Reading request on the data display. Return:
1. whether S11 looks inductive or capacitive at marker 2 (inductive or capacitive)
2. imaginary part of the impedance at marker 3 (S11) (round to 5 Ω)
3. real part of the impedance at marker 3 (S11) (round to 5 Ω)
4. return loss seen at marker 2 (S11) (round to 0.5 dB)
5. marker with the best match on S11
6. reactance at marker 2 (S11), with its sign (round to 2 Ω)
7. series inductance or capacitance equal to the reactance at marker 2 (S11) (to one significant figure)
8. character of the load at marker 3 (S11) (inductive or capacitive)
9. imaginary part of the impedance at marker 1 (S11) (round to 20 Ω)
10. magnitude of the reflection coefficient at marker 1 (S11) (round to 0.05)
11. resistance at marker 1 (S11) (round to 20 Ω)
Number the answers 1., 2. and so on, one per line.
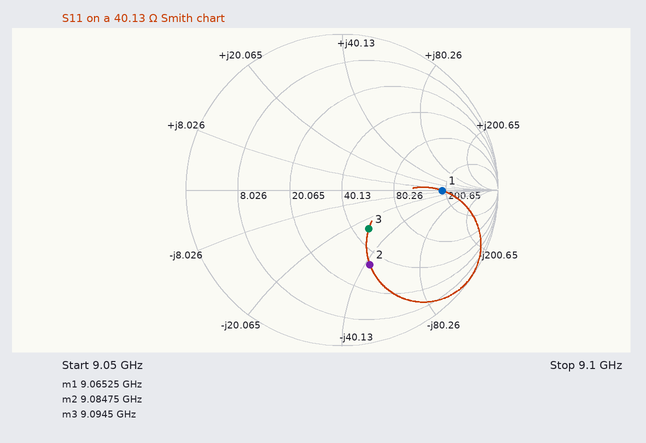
1. capacitive
2. -25 Ω
3. 50 Ω
4. 6.0 dB
5. marker 3
6. -42 Ω
7. 400 fF
8. capacitive
9. 0 Ω
10. 0.65
11. 180 Ω
